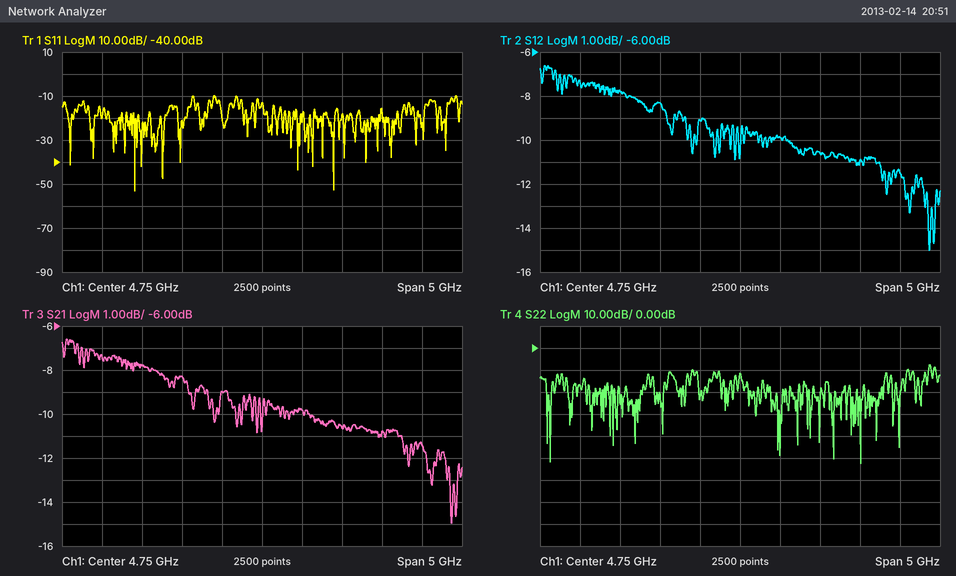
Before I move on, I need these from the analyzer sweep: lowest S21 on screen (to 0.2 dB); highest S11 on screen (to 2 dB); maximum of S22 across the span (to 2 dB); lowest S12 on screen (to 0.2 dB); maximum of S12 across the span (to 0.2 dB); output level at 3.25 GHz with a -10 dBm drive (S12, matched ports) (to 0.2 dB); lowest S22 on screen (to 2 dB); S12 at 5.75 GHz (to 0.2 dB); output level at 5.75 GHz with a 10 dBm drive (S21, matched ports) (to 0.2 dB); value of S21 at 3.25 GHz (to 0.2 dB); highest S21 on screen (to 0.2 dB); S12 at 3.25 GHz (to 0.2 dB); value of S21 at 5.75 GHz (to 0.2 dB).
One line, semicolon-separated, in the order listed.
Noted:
-15.0 dB; -10 dB; -8 dB; -15.0 dB; -6.6 dB; -17.8 dBm; -52 dB; -10.6 dB; -0.6 dBm; -7.8 dB; -6.6 dB; -7.8 dB; -10.6 dB
